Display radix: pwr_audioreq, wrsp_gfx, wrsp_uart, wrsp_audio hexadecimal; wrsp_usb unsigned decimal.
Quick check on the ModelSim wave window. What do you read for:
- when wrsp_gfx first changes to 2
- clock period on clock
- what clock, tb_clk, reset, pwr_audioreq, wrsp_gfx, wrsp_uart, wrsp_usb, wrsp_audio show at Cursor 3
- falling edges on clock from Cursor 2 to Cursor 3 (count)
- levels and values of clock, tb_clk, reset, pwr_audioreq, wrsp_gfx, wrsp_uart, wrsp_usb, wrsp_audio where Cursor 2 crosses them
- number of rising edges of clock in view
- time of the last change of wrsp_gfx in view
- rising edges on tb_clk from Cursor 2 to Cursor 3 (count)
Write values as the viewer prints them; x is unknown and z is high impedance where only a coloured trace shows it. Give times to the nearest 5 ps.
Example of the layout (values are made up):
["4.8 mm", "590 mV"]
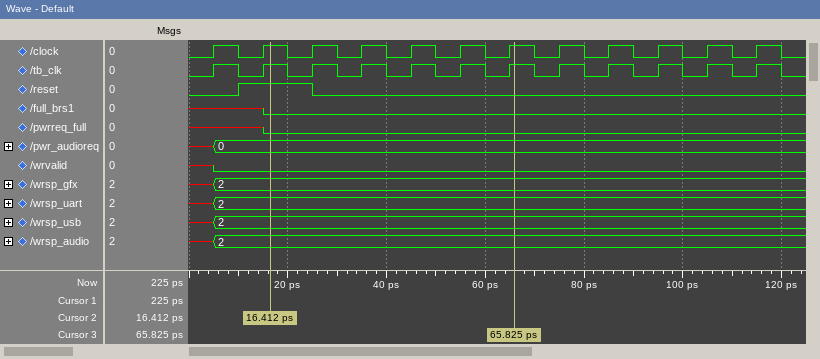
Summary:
["5 ps", "10 ps", "clock=1, tb_clk=1, reset=0, pwr_audioreq=0, wrsp_gfx=2, wrsp_uart=2, wrsp_usb=2, wrsp_audio=2", "5", "clock=1, tb_clk=1, reset=1, pwr_audioreq=0, wrsp_gfx=2, wrsp_uart=2, wrsp_usb=2, wrsp_audio=2", "12", "5 ps", "5"]
